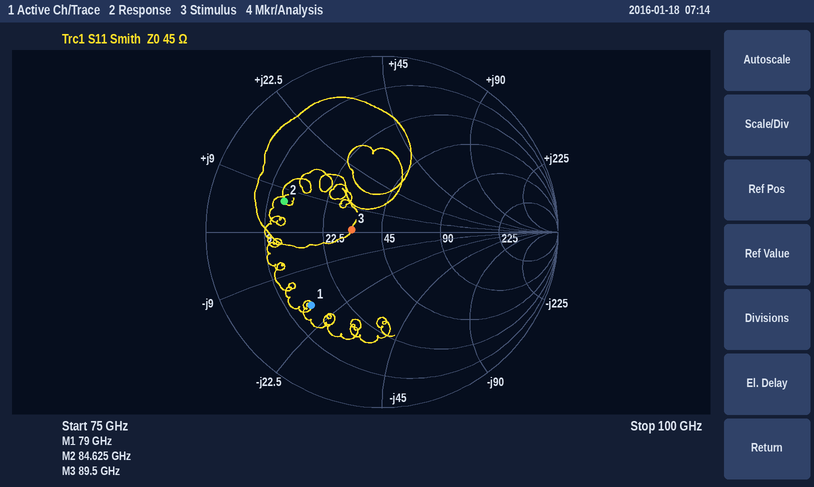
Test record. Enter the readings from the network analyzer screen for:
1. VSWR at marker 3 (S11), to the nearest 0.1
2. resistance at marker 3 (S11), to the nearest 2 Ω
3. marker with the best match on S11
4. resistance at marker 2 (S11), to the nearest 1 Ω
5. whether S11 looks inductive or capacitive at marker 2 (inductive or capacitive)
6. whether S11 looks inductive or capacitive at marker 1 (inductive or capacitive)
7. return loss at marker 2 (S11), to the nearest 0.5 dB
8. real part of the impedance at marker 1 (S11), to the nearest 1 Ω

1.4
32 Ω
marker 3
12 Ω
inductive
capacitive
4.5 dB
14 Ω
